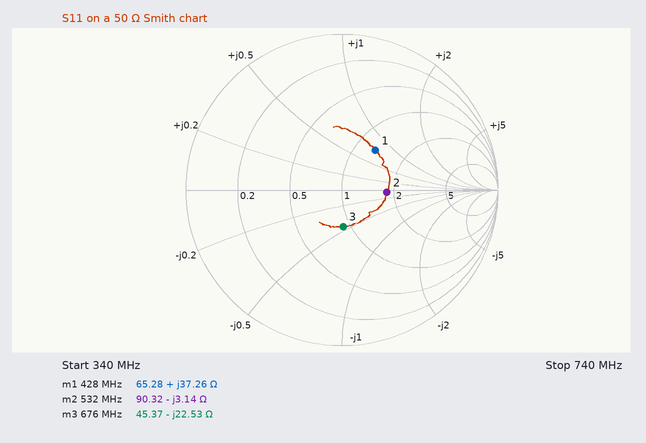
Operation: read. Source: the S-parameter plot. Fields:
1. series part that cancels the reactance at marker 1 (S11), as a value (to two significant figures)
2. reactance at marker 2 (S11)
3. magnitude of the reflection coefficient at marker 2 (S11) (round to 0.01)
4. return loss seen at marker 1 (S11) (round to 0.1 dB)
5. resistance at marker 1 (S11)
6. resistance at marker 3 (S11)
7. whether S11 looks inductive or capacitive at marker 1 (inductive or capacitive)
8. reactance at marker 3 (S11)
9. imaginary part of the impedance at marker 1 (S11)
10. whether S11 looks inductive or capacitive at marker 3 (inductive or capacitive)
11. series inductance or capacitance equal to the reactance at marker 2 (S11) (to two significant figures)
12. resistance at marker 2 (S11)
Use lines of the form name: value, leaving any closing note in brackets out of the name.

series part that cancels the reactance at marker 1 (S11), as a value: 10.0 pF
reactance at marker 2: -3.14 Ω
magnitude of the reflection coefficient at marker 2 (S11): 0.29
return loss seen at marker 1 (S11): 9.6 dB
resistance at marker 1: 65.28 Ω
resistance at marker 3: 45.37 Ω
whether S11 looks inductive or capacitive at marker 1: inductive
reactance at marker 3: -22.53 Ω
imaginary part of the impedance at marker 1: +37.26 Ω
whether S11 looks inductive or capacitive at marker 3: capacitive
series inductance or capacitance equal to the reactance at marker 2 (S11): 95 pF
resistance at marker 2: 90.32 Ω
